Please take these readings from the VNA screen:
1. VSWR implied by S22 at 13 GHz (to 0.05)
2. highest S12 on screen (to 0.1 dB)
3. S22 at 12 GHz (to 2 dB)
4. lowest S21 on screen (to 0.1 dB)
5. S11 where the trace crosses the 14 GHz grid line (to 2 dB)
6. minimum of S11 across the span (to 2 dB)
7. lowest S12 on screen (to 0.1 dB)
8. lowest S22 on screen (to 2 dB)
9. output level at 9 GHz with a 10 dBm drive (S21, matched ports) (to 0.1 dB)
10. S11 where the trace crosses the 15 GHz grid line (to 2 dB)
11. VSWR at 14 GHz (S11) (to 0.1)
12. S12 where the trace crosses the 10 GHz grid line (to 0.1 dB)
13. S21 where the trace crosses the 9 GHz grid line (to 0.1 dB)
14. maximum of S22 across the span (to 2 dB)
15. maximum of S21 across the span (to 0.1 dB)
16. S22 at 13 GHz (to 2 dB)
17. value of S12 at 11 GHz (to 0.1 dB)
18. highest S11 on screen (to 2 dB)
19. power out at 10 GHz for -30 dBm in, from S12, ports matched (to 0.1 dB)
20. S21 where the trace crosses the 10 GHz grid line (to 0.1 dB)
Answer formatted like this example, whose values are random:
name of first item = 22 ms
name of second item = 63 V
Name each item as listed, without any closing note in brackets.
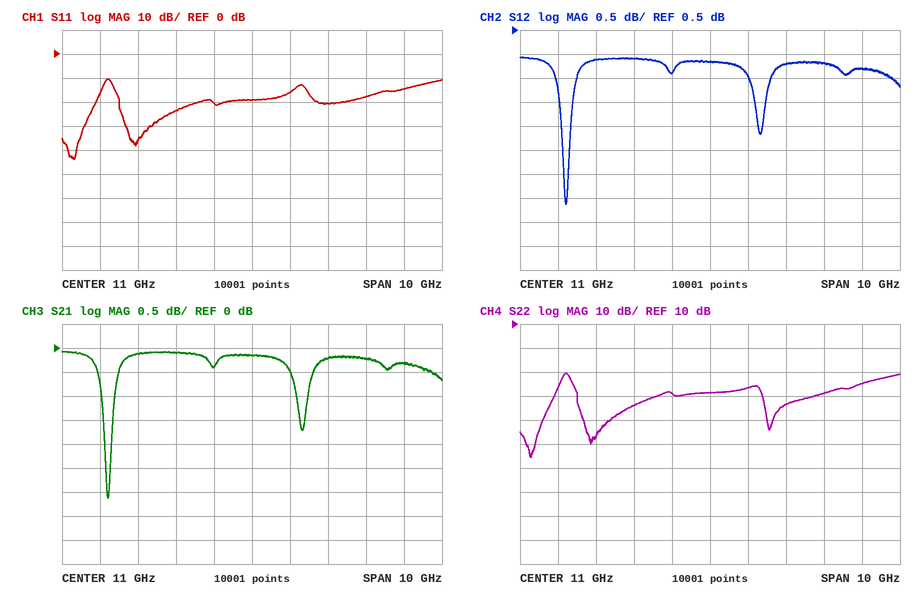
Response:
VSWR implied by S22 at 13 GHz = 1.15
highest S12 on screen = -0.1 dB
S22 at 12 GHz = -16 dB
lowest S21 on screen = -3.1 dB
S11 where the trace crosses the 14 GHz grid line = -18 dB
minimum of S11 across the span = -44 dB
lowest S12 on screen = -3.1 dB
lowest S22 on screen = -46 dB
output level at 9 GHz with a 10 dBm drive (S21, matched ports) = 9.9 dBm
S11 where the trace crosses the 15 GHz grid line = -14 dB
VSWR at 14 GHz (S11) = 1.3
S12 where the trace crosses the 10 GHz grid line = -0.4 dB
S21 where the trace crosses the 9 GHz grid line = -0.1 dB
maximum of S22 across the span = -10 dB
maximum of S21 across the span = -0.1 dB
S22 at 13 GHz = -24 dB
value of S12 at 11 GHz = -0.2 dB
highest S11 on screen = -10 dB
power out at 10 GHz for -30 dBm in, from S12, ports matched = -30.4 dBm
S21 where the trace crosses the 10 GHz grid line = -0.4 dB
